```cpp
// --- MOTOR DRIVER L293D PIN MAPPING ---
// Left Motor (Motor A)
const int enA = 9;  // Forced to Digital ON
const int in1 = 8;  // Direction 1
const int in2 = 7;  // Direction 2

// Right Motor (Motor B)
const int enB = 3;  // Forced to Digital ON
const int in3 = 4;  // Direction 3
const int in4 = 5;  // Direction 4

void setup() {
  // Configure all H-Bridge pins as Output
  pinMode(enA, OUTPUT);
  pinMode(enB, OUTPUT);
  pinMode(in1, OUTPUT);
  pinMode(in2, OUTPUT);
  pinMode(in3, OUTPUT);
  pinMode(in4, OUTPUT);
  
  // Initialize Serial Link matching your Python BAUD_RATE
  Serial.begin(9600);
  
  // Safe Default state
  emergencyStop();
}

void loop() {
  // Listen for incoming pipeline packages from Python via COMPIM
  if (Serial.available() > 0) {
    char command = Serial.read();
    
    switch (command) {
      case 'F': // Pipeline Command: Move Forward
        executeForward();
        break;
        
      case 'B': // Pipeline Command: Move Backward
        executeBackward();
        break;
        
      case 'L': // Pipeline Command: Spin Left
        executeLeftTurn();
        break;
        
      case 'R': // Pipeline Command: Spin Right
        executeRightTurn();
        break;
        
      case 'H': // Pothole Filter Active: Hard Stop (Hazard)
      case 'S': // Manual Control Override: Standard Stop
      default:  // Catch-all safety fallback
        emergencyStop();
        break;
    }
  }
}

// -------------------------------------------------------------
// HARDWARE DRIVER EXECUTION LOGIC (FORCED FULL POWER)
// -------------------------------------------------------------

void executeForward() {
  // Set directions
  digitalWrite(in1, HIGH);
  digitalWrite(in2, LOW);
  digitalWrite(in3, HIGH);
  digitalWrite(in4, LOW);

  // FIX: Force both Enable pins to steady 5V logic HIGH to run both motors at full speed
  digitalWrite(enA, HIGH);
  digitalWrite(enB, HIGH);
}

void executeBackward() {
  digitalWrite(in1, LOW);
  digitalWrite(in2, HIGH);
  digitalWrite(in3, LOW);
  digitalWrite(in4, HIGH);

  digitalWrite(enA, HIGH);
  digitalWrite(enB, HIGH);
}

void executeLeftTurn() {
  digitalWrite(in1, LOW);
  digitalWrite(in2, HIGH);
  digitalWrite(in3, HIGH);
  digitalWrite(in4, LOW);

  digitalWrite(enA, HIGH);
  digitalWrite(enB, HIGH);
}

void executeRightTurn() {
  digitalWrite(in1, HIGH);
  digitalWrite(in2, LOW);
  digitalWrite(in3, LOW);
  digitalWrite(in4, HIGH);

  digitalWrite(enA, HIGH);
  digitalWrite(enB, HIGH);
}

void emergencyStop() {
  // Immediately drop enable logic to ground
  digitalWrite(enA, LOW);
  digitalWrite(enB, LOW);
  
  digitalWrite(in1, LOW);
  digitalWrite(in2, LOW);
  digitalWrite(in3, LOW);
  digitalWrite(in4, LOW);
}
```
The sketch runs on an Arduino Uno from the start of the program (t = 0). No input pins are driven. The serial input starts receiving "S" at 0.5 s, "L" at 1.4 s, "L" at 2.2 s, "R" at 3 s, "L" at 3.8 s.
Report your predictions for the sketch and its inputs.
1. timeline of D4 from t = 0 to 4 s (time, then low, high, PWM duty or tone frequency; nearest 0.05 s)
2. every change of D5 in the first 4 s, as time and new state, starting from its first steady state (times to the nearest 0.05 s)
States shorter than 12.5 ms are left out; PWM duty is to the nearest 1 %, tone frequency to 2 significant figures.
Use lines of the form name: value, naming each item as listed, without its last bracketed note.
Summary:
timeline of D4 from t = 0 to 4 s: 0 s low; 1.4 s high; 3 s low; 3.8 s high
every change of D5 in the first 4 s, as time and new state, starting from its first steady state: 0 s low; 3 s high; 3.8 s low
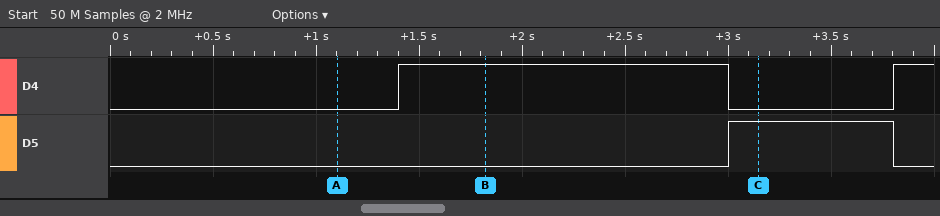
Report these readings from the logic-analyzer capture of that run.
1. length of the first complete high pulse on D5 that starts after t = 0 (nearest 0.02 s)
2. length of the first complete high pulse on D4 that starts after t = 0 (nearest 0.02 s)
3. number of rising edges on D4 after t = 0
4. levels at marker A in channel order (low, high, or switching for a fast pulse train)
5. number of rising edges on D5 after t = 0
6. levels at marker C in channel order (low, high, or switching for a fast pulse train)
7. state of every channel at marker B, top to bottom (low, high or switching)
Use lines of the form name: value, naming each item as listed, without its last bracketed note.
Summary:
length of the first complete high pulse on D5 that starts after t = 0: 0.80 s
length of the first complete high pulse on D4 that starts after t = 0: 1.60 s
number of rising edges on D4 after t = 0: 2
levels at marker A in channel order: D4 low, D5 low
number of rising edges on D5 after t = 0: 1
levels at marker C in channel order: D4 low, D5 high
state of every channel at marker B, top to bottom: D4 high, D5 low
